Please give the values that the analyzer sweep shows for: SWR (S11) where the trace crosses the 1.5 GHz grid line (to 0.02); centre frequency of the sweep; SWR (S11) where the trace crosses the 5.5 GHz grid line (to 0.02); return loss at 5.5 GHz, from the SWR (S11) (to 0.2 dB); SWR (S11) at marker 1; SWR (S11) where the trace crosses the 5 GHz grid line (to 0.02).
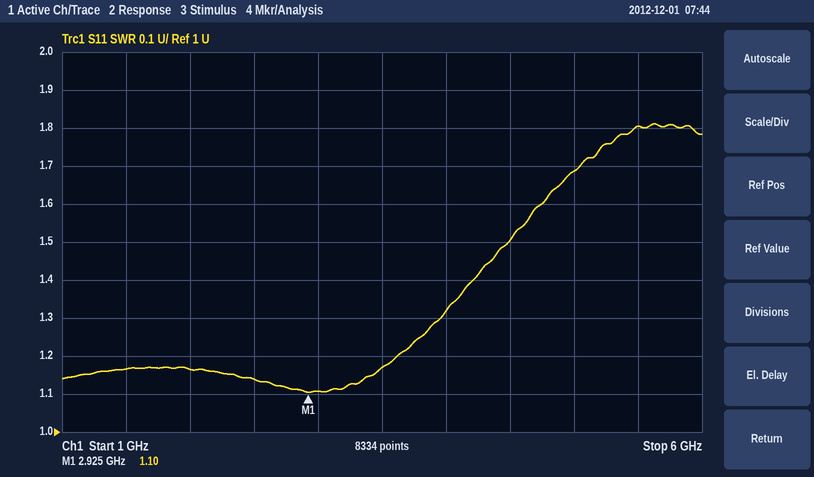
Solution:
1.16
3.5 GHz
1.80
10.8 dB
1.10
1.68
